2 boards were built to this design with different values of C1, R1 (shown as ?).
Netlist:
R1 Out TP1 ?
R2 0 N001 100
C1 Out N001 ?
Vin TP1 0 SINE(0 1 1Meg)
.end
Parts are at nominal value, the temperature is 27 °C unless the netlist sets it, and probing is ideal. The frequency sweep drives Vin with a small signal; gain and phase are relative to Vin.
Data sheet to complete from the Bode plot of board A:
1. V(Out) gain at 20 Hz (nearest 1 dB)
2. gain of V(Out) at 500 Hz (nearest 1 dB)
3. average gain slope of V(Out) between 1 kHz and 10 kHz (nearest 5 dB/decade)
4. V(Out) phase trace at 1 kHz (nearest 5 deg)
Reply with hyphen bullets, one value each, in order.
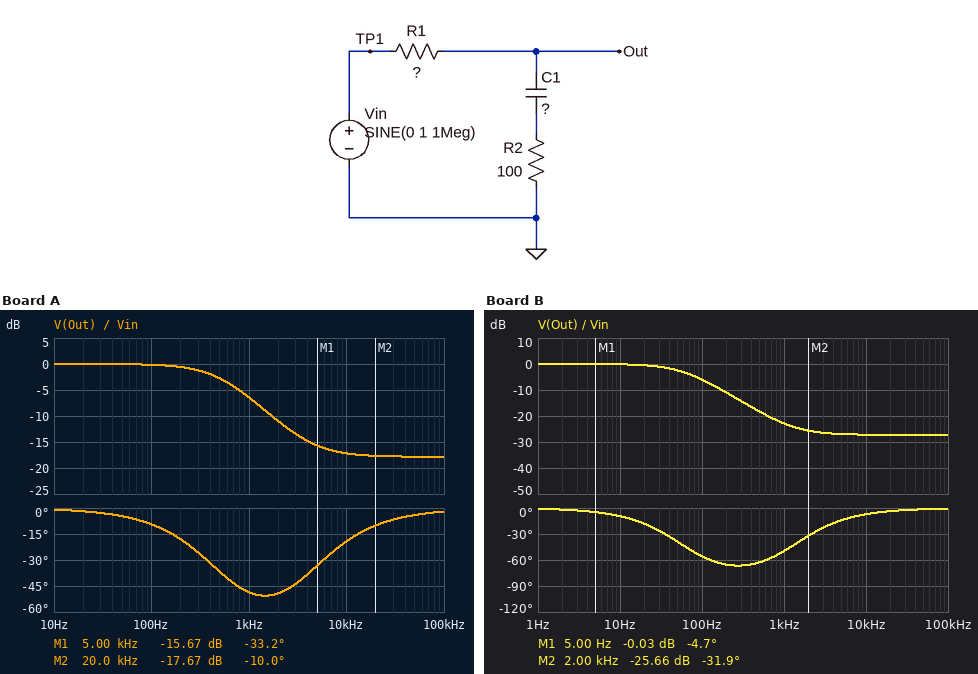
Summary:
- 0 dB
- -3 dB
- -10 dB/decade
- -50 deg
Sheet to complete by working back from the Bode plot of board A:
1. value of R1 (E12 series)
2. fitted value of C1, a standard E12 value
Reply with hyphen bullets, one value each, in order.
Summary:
- 680 Ω
- 390 nF
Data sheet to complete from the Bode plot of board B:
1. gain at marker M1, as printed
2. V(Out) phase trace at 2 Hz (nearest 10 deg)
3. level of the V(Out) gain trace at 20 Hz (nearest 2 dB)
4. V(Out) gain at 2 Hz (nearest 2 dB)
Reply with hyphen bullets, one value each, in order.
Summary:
- -0.03 dB
- 0 deg
- 0 dB
- 0 dB
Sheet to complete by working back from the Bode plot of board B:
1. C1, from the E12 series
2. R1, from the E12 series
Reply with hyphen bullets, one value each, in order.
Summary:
- 1.2 µF
- 2.2 kΩ
